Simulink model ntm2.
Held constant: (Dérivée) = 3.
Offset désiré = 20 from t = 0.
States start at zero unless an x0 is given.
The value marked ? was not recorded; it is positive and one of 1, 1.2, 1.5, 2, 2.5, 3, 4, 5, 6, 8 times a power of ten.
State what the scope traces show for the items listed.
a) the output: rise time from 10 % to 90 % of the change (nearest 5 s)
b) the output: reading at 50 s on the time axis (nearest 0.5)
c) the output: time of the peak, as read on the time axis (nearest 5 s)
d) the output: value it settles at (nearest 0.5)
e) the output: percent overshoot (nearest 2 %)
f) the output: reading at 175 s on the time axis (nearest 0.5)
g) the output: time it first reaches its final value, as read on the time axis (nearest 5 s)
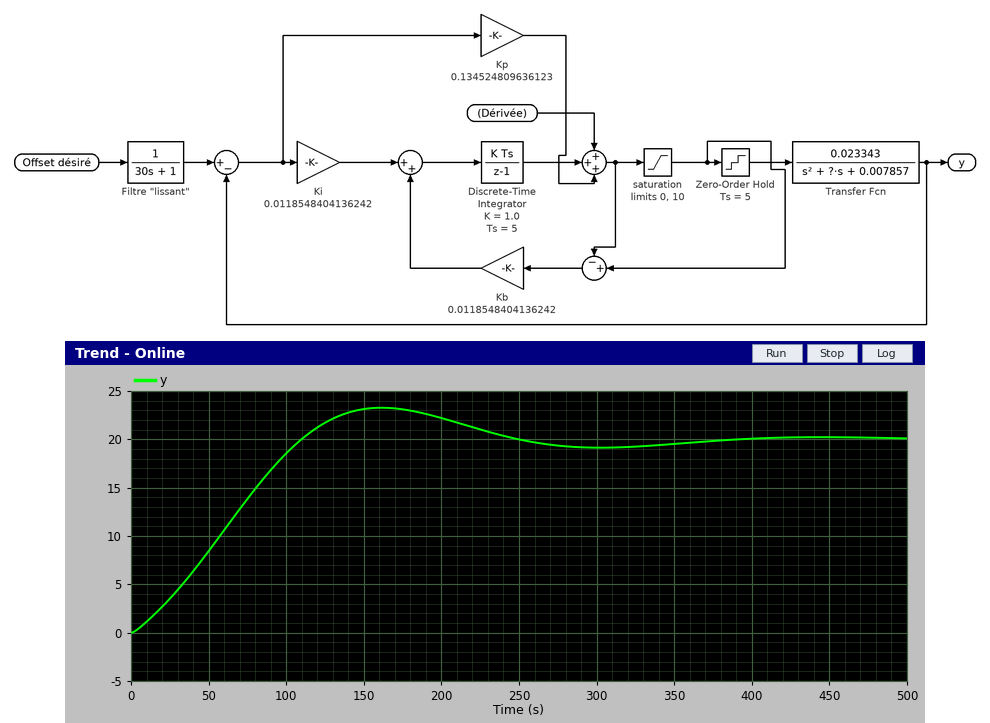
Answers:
80 s
8.5
160 s
20.0
16 %
23.0
110 s
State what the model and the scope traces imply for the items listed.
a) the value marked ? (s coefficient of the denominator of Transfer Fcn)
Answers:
0.5
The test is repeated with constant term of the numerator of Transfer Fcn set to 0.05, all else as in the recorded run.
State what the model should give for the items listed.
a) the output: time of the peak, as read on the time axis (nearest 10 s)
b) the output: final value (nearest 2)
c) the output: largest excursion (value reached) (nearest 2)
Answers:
110 s
20
22
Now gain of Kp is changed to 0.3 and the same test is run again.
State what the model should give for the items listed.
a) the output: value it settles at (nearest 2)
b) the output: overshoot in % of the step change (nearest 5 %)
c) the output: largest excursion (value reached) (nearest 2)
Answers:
20
10 %
22
